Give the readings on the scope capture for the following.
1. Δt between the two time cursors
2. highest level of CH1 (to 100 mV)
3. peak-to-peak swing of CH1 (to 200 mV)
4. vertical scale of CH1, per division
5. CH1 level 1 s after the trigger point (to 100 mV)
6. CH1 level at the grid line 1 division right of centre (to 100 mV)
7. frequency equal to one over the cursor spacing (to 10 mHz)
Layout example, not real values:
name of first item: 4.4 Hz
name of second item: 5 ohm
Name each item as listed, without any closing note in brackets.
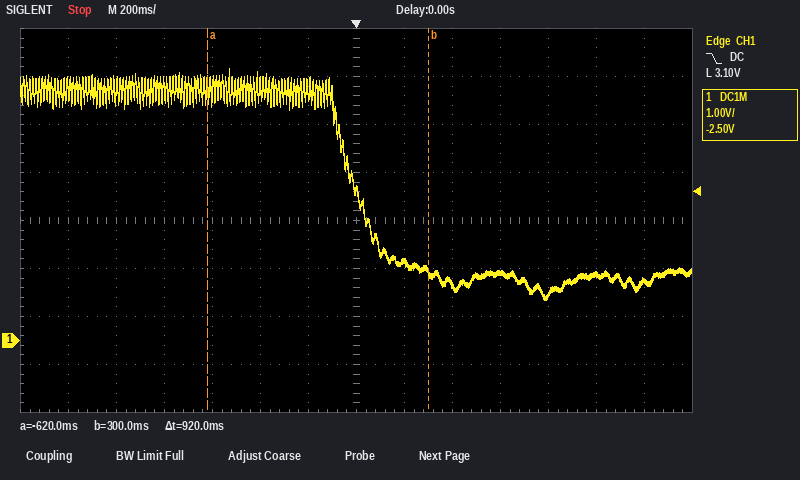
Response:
Δt between the two time cursors: 920 ms
highest level of CH1: 5.7 V
peak-to-peak swing of CH1: 4.8 V
vertical scale of CH1, per division: 1 V
CH1 level 1 s after the trigger point: 1.4 V
CH1 level at the grid line 1 division right of centre: 1.6 V
frequency equal to one over the cursor spacing: 1.09 Hz
